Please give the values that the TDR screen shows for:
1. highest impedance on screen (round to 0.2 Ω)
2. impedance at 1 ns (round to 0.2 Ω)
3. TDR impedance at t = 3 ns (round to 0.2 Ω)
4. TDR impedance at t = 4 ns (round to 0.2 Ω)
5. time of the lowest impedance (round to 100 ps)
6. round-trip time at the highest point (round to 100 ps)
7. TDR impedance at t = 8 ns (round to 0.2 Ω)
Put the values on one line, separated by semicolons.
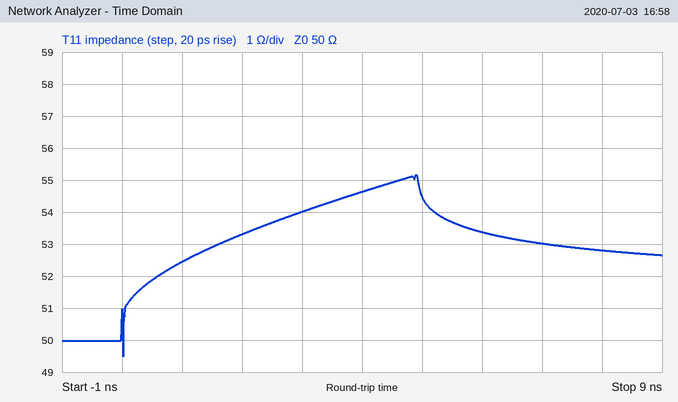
55.2 Ω; 52.4 Ω; 54.0 Ω; 54.6 Ω; 0.0 ns; 4.9 ns; 52.8 Ω
